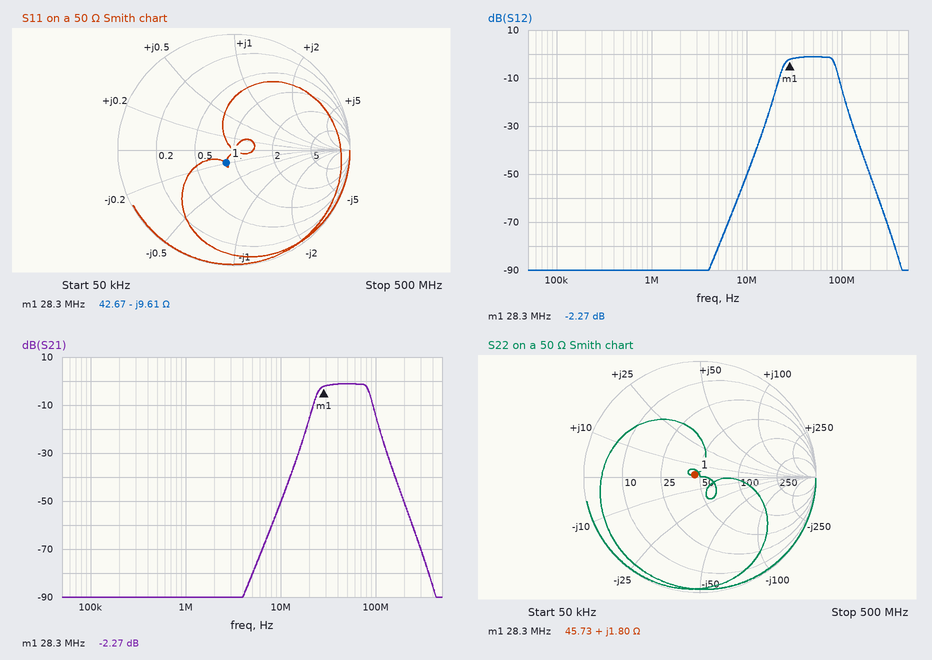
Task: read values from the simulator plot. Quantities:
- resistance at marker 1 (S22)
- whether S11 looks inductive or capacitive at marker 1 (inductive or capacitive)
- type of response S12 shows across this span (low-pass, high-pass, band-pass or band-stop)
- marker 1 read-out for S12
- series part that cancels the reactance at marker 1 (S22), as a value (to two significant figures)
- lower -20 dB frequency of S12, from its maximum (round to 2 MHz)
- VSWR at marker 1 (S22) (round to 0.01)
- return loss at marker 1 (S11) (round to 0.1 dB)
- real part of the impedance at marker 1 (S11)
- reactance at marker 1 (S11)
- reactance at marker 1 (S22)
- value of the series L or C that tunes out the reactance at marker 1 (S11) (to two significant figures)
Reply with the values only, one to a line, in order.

45.73 Ω
capacitive
band-pass
-2.27 dB
3.1 nF
18 MHz
1.10
17.7 dB
42.67 Ω
-9.61 Ω
+1.80 Ω
54 nH
